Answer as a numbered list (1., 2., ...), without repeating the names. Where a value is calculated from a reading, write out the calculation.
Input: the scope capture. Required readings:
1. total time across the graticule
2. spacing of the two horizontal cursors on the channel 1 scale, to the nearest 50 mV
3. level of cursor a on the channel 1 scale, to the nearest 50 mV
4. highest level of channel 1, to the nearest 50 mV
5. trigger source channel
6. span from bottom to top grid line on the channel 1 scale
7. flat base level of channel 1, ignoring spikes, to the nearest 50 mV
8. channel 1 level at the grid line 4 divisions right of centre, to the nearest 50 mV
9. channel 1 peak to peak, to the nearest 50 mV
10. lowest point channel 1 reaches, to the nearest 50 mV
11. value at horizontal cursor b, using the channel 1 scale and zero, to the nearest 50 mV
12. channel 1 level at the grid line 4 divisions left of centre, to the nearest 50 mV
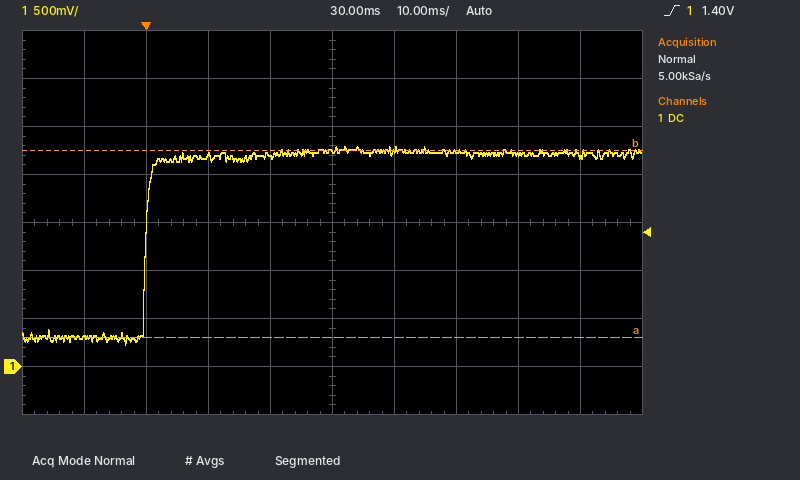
1. 100 ms
2. 1.95 V
3. 300 mV
4. 2.30 V
5. channel 1
6. 4 V
7. 300 mV
8. 2.20 V
9. 2.30 V − (250 mV) = 2.05 V
10. 250 mV
11. 2.25 V
12. 300 mV
